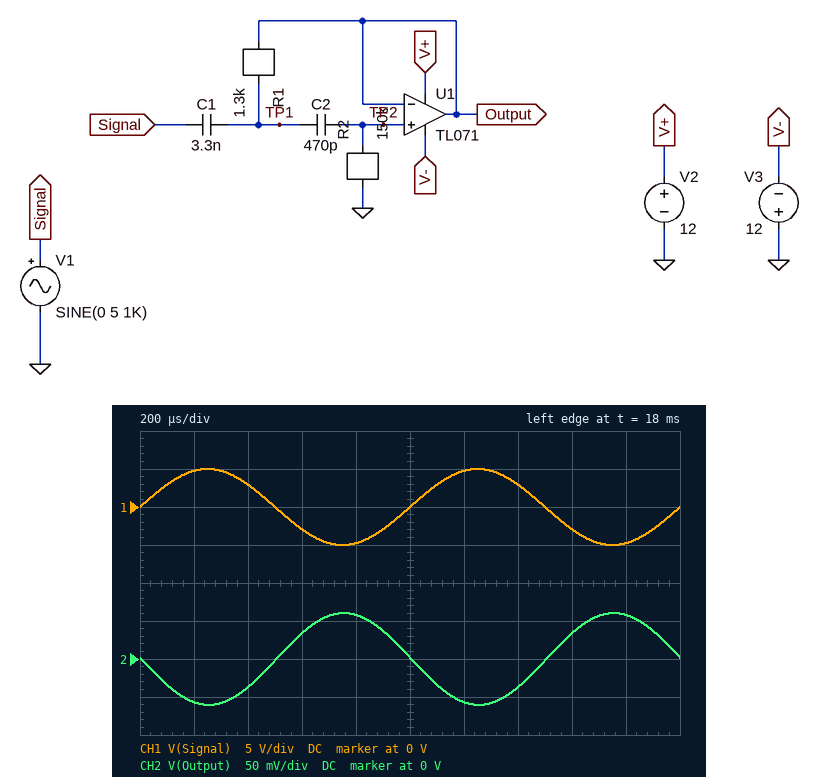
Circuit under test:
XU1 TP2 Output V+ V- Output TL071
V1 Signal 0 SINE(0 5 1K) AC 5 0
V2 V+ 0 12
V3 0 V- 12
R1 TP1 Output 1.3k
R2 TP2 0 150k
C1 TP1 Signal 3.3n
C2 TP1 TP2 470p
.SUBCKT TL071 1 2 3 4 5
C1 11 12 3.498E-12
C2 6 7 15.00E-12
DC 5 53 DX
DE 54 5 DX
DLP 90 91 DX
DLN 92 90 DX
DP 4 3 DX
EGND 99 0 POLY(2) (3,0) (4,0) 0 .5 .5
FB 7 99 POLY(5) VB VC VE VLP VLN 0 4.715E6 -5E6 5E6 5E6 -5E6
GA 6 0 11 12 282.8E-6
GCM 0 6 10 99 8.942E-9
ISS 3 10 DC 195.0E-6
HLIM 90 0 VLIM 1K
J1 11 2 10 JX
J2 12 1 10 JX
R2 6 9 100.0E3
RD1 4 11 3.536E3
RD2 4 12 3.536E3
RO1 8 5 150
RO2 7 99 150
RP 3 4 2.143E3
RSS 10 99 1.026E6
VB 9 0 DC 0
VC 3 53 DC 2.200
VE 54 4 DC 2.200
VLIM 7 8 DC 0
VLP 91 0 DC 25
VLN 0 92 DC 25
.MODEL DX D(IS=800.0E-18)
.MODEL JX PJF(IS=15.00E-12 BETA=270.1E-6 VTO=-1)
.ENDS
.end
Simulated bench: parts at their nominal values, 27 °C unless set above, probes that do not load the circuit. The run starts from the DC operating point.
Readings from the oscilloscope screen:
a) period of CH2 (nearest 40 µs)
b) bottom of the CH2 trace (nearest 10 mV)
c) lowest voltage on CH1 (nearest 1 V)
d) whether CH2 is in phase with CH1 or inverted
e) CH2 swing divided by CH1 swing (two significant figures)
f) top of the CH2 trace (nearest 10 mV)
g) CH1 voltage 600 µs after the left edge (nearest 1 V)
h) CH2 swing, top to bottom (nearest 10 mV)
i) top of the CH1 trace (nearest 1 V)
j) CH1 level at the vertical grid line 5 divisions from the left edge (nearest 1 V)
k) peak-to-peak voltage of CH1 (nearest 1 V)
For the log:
1.00 ms
-60 mV
-5 V
inverted
0.012
60 mV
-3 V
120 mV
5 V
0 V
10 V
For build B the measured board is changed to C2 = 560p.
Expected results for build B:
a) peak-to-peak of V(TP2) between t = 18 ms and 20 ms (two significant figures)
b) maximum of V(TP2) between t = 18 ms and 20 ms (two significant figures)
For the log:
140 mV
72 mV
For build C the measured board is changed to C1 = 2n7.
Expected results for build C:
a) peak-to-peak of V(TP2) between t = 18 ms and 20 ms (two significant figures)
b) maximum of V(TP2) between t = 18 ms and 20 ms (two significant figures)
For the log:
99 mV
49 mV
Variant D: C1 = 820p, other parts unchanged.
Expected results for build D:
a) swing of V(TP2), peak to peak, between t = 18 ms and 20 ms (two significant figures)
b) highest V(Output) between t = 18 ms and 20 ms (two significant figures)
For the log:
30 mV
15 mV
